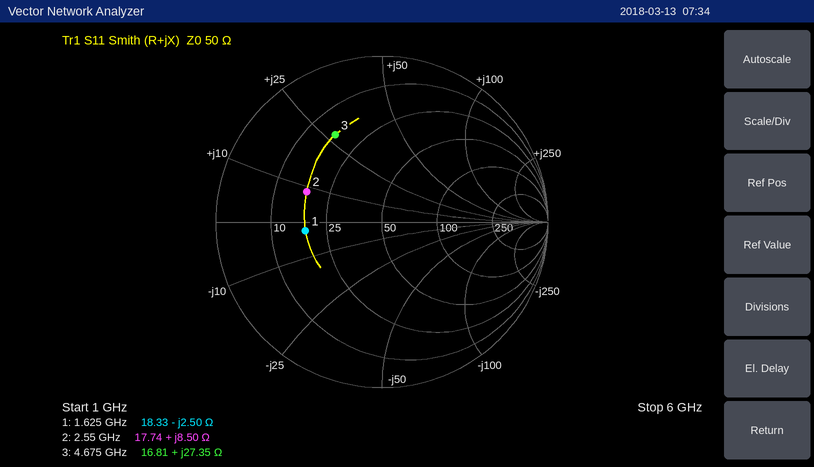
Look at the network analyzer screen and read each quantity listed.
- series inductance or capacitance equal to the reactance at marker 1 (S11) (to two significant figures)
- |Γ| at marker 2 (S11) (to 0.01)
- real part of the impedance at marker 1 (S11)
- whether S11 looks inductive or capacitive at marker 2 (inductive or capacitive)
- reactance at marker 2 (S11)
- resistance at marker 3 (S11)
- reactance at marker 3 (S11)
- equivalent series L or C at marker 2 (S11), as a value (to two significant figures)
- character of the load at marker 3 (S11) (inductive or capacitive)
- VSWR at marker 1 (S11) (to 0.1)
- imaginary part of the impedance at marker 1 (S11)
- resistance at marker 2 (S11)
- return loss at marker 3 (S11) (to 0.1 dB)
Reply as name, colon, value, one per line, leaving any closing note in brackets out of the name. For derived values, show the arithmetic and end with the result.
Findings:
series inductance or capacitance equal to the reactance at marker 1 (S11): C = 1/(2π × 1.625 GHz × 2.5 Ω) ≈ 39 pF
|Γ| at marker 2 (S11): 0.49
real part of the impedance at marker 1: 18.33 Ω
whether S11 looks inductive or capacitive at marker 2: inductive
reactance at marker 2: +8.50 Ω
resistance at marker 3: 16.81 Ω
reactance at marker 3: +27.35 Ω
equivalent series L or C at marker 2 (S11), as a value: L = 8.5 Ω/(2π × 2.55 GHz) ≈ 531 pH, so 530 pH to two significant figures
character of the load at marker 3 (S11): inductive
VSWR at marker 1 (S11): 2.7
imaginary part of the impedance at marker 1: -2.50 Ω
resistance at marker 2: 17.74 Ω
return loss at marker 3 (S11): 4.5 dB
